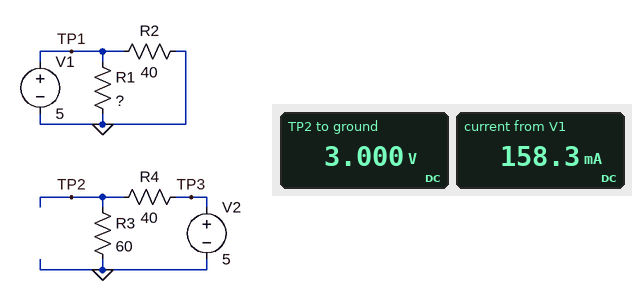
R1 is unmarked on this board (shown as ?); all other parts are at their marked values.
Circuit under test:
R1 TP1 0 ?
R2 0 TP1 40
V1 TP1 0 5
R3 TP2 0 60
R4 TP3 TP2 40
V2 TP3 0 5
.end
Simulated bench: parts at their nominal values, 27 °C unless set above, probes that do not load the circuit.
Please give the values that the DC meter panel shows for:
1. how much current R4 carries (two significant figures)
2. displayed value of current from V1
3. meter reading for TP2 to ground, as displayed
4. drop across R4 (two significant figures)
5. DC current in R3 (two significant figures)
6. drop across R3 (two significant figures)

50 mA
158.3 mA
3.000 V
2.0 V
50 mA
3.0 V
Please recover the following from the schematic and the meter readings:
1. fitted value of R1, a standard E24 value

150 Ω
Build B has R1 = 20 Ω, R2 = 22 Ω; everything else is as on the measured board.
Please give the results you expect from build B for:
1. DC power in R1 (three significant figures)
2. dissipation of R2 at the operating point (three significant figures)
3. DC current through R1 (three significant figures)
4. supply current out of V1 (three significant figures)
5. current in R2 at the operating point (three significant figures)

1.25 W
1.14 W
250 mA
477 mA
227 mA
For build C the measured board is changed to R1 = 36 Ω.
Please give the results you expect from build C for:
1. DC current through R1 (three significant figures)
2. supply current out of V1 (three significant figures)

139 mA
264 mA
